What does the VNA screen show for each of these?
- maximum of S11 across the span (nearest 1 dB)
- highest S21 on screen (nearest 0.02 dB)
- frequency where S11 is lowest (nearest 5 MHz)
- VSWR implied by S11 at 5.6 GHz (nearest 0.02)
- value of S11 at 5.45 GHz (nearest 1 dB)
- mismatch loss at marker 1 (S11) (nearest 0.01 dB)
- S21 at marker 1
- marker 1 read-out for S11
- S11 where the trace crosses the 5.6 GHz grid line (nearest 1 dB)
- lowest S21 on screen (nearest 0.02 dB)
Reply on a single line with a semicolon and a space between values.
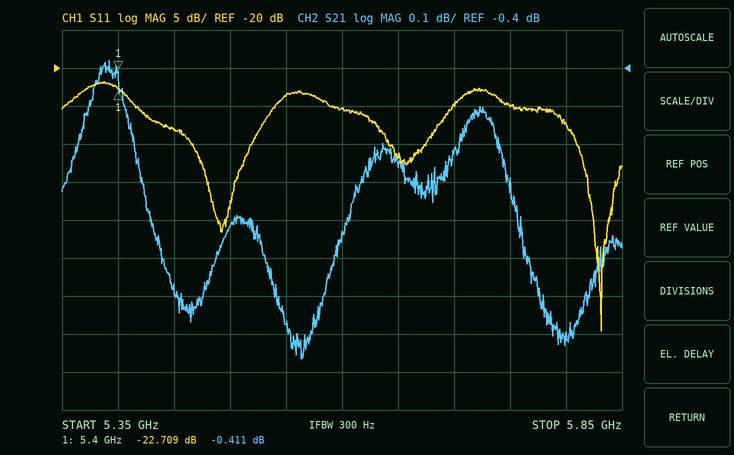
-22 dB; -0.38 dB; 5.830 GHz; 1.12; -28 dB; 0.02 dB; -0.411 dB; -22.709 dB; -25 dB; -1.16 dB
